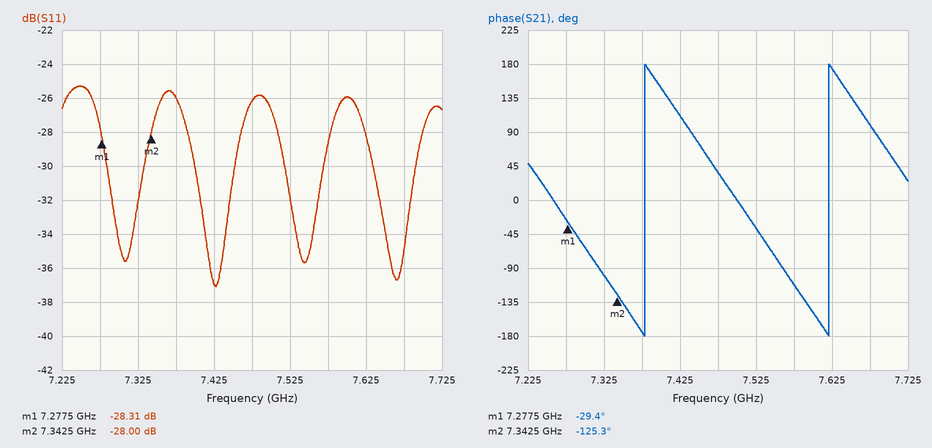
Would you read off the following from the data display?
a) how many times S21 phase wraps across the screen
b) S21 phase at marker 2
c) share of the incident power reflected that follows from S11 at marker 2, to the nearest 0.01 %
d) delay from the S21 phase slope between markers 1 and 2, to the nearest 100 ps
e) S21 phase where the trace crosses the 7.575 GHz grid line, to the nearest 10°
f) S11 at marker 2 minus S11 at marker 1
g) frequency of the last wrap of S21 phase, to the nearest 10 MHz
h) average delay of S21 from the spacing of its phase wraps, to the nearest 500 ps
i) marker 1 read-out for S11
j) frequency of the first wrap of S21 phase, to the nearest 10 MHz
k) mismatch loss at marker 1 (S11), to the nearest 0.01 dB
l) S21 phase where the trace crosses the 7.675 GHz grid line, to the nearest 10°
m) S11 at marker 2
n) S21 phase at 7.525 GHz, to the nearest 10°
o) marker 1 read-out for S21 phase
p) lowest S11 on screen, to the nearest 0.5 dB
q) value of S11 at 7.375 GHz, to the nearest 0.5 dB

2
-125.3°
0.16 %
4.1 ns
-110°
0.31 dB
7.62 GHz
4.0 ns
-28.31 dB
7.38 GHz
0.01 dB
100°
-28.00 dB
-40°
-29.4°
-37.0 dB
-26.0 dB
